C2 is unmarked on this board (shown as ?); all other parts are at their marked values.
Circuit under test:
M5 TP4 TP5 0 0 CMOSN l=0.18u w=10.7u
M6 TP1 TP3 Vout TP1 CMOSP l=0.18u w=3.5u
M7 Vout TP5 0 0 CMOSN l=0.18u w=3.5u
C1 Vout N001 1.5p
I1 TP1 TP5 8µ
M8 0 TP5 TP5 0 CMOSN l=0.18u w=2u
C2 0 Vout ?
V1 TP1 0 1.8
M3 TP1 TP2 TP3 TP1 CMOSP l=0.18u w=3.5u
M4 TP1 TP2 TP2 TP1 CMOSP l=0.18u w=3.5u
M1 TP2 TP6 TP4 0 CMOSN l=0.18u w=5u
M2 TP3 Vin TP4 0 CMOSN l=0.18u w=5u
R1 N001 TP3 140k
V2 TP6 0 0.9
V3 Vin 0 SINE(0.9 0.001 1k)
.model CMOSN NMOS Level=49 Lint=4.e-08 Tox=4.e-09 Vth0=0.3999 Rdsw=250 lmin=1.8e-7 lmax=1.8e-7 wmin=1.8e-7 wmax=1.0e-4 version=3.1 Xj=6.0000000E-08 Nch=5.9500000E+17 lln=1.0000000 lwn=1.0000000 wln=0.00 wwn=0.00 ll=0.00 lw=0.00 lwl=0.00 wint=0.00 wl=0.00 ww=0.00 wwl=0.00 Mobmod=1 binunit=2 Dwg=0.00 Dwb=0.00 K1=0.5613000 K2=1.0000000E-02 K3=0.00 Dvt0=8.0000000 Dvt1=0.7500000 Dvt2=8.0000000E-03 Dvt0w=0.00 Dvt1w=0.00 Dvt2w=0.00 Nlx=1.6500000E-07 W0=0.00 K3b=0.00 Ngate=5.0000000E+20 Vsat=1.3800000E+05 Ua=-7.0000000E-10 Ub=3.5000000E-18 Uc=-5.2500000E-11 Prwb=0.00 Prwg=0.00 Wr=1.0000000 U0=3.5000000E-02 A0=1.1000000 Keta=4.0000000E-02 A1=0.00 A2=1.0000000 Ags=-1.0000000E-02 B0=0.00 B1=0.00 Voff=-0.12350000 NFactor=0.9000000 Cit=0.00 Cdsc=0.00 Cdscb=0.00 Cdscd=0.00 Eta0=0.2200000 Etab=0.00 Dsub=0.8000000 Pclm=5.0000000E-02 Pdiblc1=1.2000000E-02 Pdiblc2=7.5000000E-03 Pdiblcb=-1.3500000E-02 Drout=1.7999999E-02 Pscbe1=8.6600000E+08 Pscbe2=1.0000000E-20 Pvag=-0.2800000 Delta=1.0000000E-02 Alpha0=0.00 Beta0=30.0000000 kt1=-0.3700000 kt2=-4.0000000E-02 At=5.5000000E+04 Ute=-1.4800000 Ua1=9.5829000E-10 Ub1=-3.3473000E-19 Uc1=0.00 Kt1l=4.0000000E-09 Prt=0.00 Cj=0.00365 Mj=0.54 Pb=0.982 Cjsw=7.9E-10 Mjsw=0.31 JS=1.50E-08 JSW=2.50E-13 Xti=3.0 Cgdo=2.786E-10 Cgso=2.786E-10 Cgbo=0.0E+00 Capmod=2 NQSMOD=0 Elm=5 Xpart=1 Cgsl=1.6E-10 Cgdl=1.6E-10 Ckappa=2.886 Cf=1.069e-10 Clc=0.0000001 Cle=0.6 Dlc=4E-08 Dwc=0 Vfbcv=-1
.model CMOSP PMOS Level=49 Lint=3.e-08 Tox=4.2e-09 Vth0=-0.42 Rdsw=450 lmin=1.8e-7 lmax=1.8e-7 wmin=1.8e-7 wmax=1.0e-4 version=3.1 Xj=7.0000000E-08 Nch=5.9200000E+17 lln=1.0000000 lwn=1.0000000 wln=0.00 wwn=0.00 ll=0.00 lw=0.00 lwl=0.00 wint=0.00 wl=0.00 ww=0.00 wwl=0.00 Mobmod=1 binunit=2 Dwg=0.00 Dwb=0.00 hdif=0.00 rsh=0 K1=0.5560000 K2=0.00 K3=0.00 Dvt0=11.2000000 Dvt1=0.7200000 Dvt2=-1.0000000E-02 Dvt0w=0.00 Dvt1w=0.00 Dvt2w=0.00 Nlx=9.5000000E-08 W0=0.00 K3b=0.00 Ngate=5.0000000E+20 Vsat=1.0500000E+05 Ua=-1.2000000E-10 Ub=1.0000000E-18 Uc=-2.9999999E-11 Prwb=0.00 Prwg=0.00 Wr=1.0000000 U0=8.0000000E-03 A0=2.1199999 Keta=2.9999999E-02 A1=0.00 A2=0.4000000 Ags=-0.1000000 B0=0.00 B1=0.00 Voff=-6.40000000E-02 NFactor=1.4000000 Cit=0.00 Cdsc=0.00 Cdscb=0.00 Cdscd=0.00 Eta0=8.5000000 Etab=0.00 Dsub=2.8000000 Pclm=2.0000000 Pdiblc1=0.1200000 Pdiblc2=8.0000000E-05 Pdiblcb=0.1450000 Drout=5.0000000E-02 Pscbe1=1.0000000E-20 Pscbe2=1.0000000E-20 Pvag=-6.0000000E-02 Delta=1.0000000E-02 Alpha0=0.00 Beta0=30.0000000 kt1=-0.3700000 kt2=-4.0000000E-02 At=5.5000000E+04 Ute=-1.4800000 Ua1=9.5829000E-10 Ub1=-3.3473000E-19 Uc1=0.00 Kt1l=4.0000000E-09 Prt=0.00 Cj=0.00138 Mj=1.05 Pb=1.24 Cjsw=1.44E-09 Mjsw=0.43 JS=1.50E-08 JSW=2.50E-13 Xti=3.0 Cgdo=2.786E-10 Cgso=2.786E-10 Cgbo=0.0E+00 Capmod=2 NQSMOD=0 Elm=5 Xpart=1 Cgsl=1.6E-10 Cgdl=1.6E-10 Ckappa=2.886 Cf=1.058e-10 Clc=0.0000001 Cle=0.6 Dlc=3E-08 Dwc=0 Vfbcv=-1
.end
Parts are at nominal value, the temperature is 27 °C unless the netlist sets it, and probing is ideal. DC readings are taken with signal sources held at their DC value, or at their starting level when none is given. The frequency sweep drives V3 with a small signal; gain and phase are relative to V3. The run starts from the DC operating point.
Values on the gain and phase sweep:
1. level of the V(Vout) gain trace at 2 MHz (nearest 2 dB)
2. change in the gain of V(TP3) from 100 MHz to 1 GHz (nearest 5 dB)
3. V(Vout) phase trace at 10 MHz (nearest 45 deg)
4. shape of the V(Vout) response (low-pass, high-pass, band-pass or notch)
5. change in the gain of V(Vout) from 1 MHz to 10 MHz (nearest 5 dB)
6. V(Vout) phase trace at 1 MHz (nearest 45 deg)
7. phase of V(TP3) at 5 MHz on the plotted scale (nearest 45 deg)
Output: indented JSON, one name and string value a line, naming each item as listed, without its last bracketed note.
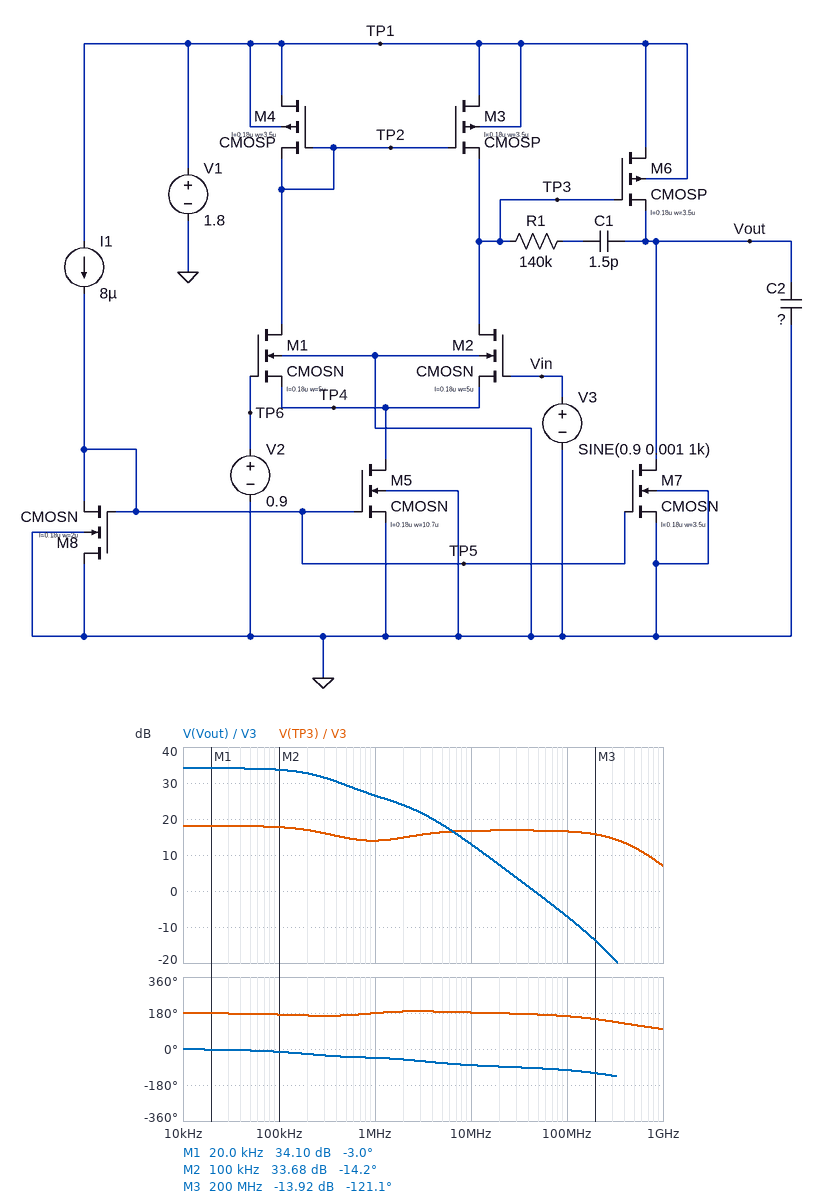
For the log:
{
  "level of the V(Vout) gain trace at 2 MHz": "24 dB",
  "change in the gain of V(TP3) from 100 MHz to 1 GHz": "-10 dB",
  "V(Vout) phase trace at 10 MHz": "-90 deg",
  "shape of the V(Vout) response": "low-pass",
  "change in the gain of V(Vout) from 1 MHz to 10 MHz": "-15 dB",
  "V(Vout) phase trace at 1 MHz": "-45 deg",
  "phase of V(TP3) at 5 MHz on the plotted scale": "180 deg"
}
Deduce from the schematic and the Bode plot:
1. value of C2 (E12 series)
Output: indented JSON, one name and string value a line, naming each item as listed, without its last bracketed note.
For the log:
{
  "value of C2": "8.2 pF"
}
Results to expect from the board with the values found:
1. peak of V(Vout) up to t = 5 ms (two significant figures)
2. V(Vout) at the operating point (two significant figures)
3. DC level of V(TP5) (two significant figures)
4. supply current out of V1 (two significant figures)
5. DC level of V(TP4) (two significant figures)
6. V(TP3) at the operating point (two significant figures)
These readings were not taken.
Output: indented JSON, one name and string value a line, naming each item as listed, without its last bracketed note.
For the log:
{
  "peak of V(Vout) up to t = 5 ms": "1.0 V",
  "V(Vout) at the operating point": "980 mV",
  "DC level of V(TP5)": "420 mV",
  "supply current out of V1": "83 µA",
  "DC level of V(TP4)": "450 mV",
  "V(TP3) at the operating point": "1.4 V"
}
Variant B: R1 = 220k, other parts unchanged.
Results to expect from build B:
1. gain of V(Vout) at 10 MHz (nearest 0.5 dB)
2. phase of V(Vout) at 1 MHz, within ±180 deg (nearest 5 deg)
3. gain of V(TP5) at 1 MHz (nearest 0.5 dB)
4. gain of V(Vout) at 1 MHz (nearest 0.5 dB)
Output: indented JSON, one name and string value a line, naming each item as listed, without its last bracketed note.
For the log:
{
  "gain of V(Vout) at 10 MHz": "13.5 dB",
  "phase of V(Vout) at 1 MHz, within ±180 deg": "-40 deg",
  "gain of V(TP5) at 1 MHz": "-55.5 dB",
  "gain of V(Vout) at 1 MHz": "27.5 dB"
}
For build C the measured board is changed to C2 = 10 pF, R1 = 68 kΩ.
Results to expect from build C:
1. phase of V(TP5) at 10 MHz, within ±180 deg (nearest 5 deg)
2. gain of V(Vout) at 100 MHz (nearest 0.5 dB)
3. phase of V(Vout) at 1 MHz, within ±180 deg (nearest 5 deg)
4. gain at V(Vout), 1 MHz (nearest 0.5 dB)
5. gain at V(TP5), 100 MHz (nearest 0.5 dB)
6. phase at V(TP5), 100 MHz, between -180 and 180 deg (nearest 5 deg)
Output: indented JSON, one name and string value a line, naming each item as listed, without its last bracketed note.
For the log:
{
  "phase of V(TP5) at 10 MHz, within ±180 deg": "20 deg",
  "gain of V(Vout) at 100 MHz": "-10.0 dB",
  "phase of V(Vout) at 1 MHz, within ±180 deg": "-60 deg",
  "gain at V(Vout), 1 MHz": "25.0 dB",
  "gain at V(TP5), 100 MHz": "-47.0 dB",
  "phase at V(TP5), 100 MHz, between -180 and 180 deg": "70 deg"
}
